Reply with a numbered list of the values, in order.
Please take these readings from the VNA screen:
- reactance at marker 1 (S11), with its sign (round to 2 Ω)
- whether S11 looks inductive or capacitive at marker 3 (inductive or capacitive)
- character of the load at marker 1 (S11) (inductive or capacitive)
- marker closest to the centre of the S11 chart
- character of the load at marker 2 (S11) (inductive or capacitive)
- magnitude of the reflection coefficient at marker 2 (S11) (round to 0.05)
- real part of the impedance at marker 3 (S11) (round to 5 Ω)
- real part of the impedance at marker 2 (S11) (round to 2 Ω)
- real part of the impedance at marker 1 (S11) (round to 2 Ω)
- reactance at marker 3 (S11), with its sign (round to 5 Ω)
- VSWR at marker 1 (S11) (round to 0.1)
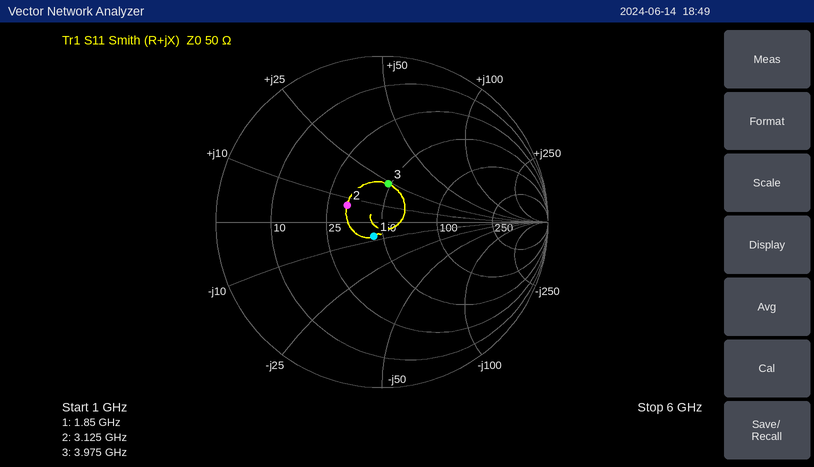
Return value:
1. -8 Ω
2. inductive
3. capacitive
4. marker 1
5. inductive
6. 0.25
7. 50 Ω
8. 32 Ω
9. 44 Ω
10. +25 Ω
11. 1.2
